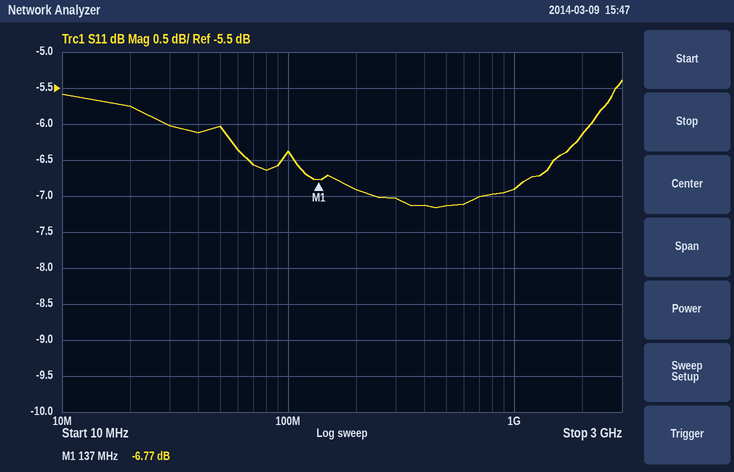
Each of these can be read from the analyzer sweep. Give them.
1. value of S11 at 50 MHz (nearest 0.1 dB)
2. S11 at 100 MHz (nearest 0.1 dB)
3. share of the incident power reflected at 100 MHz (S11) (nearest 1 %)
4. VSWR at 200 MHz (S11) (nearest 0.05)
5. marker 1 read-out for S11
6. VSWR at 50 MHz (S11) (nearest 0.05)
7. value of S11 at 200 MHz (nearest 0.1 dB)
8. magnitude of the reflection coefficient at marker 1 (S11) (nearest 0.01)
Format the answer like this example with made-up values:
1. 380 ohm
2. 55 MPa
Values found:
1. -6.0 dB
2. -6.4 dB
3. 23 %
4. 2.65
5. -6.77 dB
6. 3.00
7. -6.9 dB
8. 0.46
